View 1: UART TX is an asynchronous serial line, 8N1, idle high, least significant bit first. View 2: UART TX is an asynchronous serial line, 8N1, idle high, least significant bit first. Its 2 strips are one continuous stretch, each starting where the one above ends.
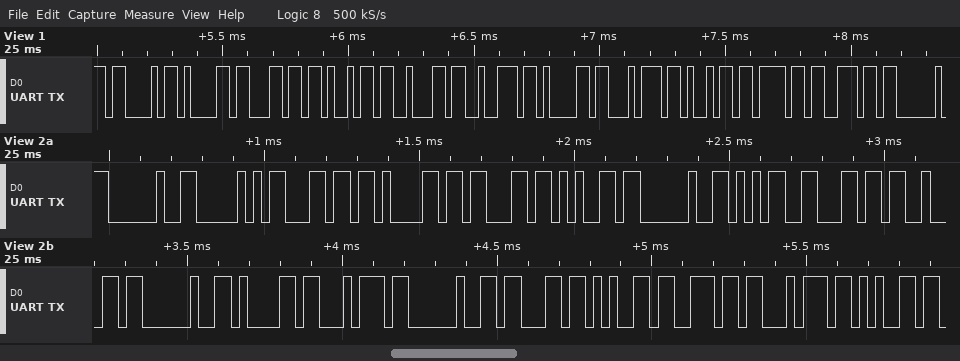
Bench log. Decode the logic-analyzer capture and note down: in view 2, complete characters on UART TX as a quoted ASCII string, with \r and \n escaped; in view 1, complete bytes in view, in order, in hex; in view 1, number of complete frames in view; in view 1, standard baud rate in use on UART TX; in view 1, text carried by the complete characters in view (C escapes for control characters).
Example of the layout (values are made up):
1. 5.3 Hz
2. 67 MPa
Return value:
1. " Place 5lb at cente"
2. 43 61 6C 69 62 72 61 74 69 6F 6E
3. 11
4. 38400 baud
5. "Calibration"
